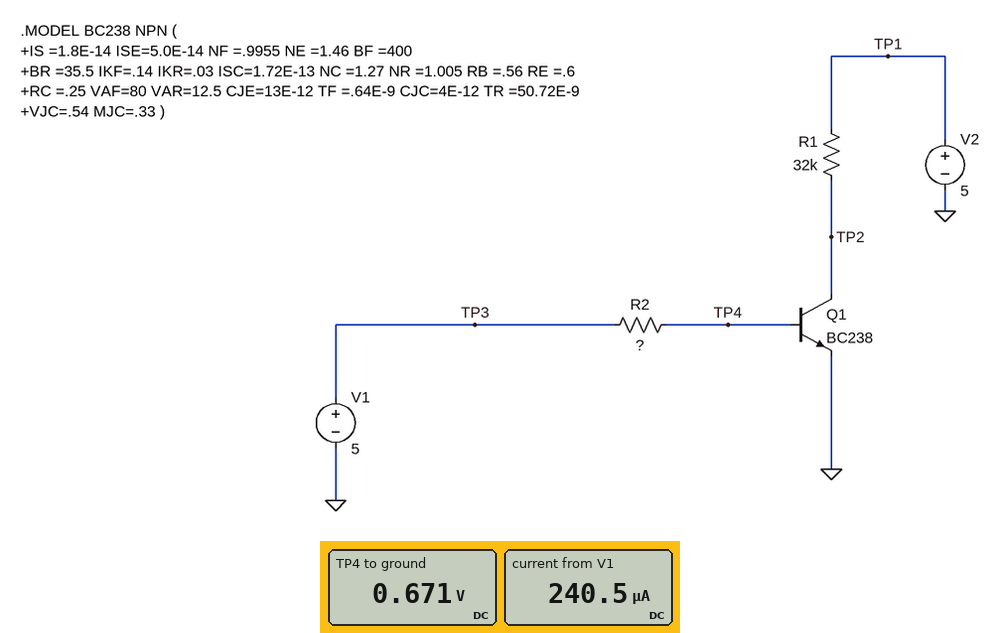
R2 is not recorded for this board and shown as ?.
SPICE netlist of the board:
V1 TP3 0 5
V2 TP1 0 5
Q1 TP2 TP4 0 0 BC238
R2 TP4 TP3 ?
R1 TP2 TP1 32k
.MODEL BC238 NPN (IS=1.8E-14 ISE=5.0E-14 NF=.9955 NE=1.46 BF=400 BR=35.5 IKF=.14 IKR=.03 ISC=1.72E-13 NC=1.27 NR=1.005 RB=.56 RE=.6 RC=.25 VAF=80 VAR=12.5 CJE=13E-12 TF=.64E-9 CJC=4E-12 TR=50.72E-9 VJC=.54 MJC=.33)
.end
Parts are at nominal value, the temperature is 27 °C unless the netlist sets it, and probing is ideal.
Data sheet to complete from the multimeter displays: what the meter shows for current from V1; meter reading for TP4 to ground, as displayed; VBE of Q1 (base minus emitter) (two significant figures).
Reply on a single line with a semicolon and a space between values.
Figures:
240.5 µA; 0.671 V; 670 mV
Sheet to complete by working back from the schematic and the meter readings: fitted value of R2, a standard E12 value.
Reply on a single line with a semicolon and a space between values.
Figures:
18 kΩ
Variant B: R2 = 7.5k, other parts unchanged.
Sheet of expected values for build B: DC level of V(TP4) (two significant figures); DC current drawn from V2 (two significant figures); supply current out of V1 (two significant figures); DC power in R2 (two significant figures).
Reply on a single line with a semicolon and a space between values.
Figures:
700 mV; 160 µA; 570 µA; 2.5 mW
